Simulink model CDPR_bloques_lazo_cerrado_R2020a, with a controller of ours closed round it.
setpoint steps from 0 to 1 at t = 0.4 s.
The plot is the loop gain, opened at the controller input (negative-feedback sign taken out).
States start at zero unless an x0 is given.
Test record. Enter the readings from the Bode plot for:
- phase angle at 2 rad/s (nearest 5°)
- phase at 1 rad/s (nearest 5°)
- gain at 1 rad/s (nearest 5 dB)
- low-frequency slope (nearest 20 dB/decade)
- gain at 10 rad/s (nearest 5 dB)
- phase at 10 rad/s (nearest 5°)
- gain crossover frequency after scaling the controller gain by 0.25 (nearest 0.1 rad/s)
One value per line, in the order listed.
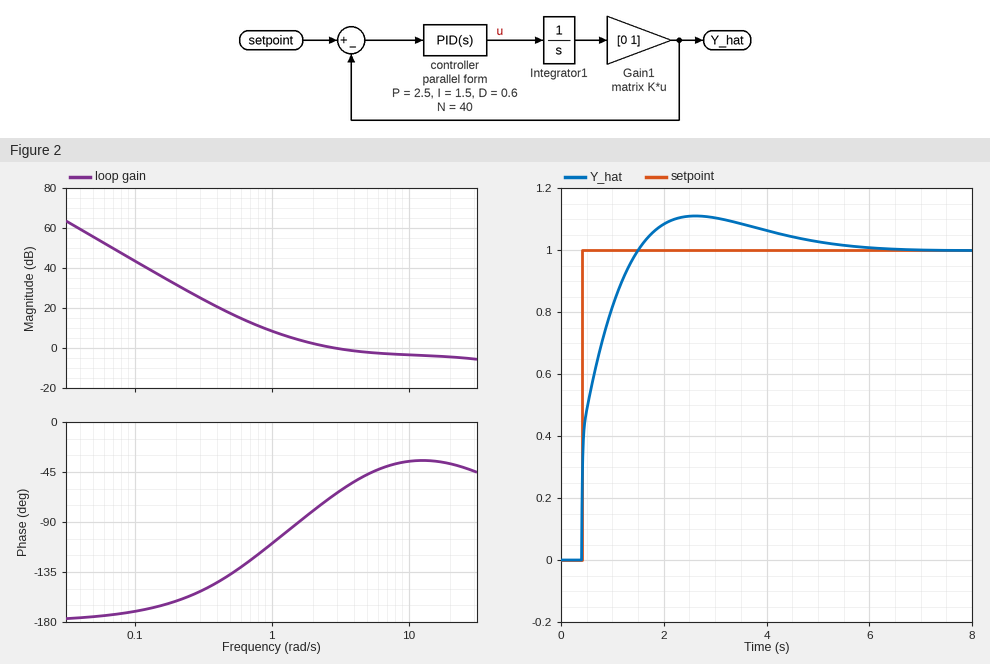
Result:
-80°
-110°
10 dB
-40 dB/decade
-5 dB
-35°
0.7 rad/s
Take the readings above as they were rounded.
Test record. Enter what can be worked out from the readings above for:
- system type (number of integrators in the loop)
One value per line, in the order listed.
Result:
2
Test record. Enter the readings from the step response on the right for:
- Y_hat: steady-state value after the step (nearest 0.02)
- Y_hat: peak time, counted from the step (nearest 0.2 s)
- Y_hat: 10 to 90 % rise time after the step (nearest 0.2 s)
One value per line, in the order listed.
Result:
1.00
2.2 s
0.8 s
